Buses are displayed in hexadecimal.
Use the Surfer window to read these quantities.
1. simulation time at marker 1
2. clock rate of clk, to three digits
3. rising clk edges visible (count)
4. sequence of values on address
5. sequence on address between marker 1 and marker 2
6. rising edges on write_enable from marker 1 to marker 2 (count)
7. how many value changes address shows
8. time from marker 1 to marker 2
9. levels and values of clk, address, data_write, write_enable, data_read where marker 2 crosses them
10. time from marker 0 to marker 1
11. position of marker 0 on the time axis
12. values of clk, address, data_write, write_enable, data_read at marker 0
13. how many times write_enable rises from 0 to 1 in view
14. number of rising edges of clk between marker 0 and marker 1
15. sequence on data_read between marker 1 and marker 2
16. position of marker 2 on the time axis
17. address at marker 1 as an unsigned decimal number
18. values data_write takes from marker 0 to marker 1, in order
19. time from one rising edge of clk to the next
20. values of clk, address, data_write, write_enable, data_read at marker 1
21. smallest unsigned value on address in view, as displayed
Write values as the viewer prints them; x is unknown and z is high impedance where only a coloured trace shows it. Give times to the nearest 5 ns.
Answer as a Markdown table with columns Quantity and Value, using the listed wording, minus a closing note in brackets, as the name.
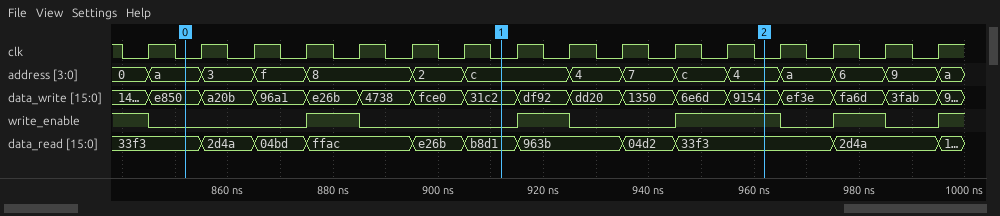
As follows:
| Quantity | Value |
|---|---|
| simulation time at marker 1 | 910 ns |
| clock rate of clk, to three digits | 100 MHz |
| rising clk edges visible | 16 |
| sequence of values on address | 0, a, 3, f, 8, 2, c, 4, 7, c, 4, a, 6, 9, a |
| sequence on address between marker 1 and marker 2 | c, 4, 7, c, 4 |
| rising edges on write_enable from marker 1 to marker 2 | 2 |
| how many value changes address shows | 14 |
| time from marker 1 to marker 2 | 50 ns |
| levels and values of clk, address, data_write, write_enable, data_read where marker 2 crosses them | clk=0, address=4, data_write=9154, write_enable=1, data_read=33f3 |
| time from marker 0 to marker 1 | 60 ns |
| position of marker 0 on the time axis | 850 ns |
| values of clk, address, data_write, write_enable, data_read at marker 0 | clk=0, address=a, data_write=e850, write_enable=0, data_read=33f3 |
| how many times write_enable rises from 0 to 1 in view | 5 |
| number of rising edges of clk between marker 0 and marker 1 | 6 |
| sequence on data_read between marker 1 and marker 2 | b8d1, 963b, 04d2, 33f3 |
| position of marker 2 on the time axis | 960 ns |
| address at marker 1 as an unsigned decimal number | 12 |
| values data_write takes from marker 0 to marker 1, in order | e850, a20b, 96a1, e26b, 4738, fce0, 31c2 |
| time from one rising edge of clk to the next | 10 ns |
| values of clk, address, data_write, write_enable, data_read at marker 1 | clk=0, address=c, data_write=31c2, write_enable=0, data_read=b8d1 |
| smallest unsigned value on address in view, as displayed | 0 |
